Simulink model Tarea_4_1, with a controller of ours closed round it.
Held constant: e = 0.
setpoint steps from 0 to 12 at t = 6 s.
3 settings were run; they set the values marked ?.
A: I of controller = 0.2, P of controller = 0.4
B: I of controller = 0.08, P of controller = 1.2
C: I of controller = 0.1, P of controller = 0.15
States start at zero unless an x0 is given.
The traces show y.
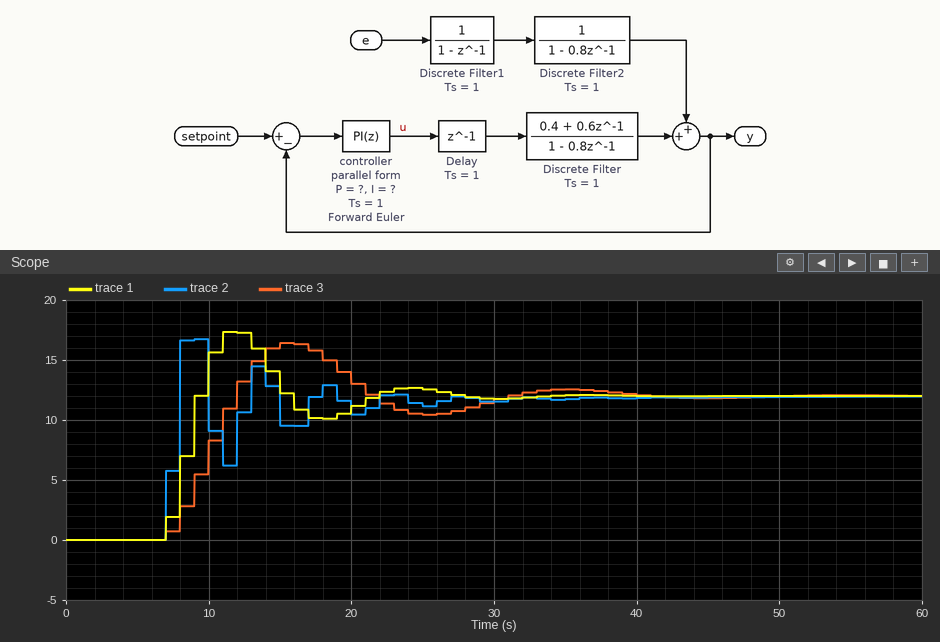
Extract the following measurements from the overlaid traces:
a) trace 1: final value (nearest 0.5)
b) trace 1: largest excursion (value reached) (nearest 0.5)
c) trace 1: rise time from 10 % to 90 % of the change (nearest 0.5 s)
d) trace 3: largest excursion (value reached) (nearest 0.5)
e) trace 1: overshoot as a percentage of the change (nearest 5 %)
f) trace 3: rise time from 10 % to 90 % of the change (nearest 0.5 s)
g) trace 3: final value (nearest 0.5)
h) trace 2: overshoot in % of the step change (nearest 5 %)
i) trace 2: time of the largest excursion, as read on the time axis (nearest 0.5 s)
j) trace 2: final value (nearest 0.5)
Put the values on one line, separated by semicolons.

12.0; 17.5; 2.0 s; 16.5; 45 %; 3.0 s; 12.0; 40 %; 9.0 s; 12.0
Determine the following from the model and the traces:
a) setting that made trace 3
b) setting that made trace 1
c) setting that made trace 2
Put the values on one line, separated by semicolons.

C; A; B
